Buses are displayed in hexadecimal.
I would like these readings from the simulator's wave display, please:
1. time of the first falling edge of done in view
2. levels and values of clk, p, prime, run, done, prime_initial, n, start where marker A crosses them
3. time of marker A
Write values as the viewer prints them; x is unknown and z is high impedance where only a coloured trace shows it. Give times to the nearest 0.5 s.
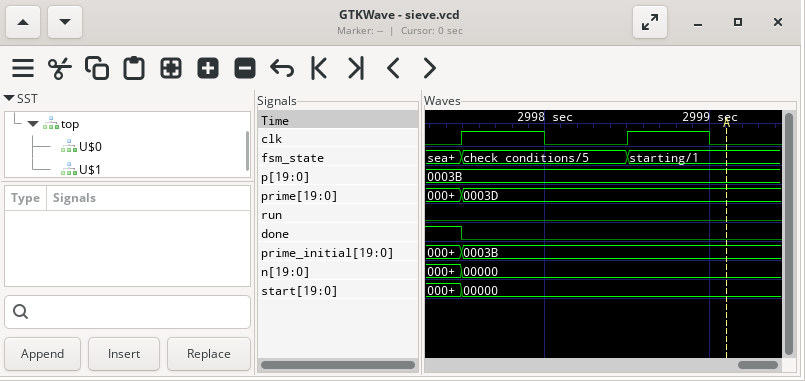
2997.5 s
clk=0, p=0003B, prime=0003D, run=0, done=0, prime_initial=0003B, n=00000, start=00000
2999 s
